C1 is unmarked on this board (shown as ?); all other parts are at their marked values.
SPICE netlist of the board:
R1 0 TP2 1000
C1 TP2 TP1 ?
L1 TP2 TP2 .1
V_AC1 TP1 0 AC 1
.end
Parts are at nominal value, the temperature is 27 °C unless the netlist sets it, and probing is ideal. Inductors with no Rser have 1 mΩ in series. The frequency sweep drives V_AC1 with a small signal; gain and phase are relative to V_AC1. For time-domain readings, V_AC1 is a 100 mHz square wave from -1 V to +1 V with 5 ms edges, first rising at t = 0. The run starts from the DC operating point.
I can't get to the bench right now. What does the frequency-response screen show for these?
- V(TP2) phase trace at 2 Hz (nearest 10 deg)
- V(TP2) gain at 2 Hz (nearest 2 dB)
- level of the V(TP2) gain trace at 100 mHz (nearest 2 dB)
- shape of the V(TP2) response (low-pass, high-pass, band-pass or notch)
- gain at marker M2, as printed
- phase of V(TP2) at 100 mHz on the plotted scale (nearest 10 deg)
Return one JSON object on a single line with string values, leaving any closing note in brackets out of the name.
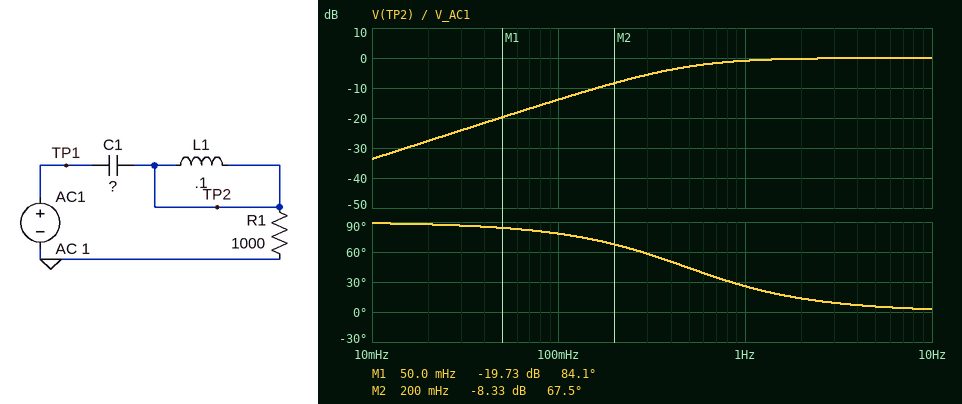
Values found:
{"V(TP2) phase trace at 2 Hz": "10 deg", "V(TP2) gain at 2 Hz": "0 dB", "level of the V(TP2) gain trace at 100 mHz": "-14 dB", "shape of the V(TP2) response": "high-pass", "gain at marker M2, as printed": "-8.33 dB", "phase of V(TP2) at 100 mHz on the plotted scale": "80 deg"}
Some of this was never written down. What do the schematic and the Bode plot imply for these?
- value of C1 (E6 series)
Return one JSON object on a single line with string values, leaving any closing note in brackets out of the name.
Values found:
{"value of C1": "330 µF"}
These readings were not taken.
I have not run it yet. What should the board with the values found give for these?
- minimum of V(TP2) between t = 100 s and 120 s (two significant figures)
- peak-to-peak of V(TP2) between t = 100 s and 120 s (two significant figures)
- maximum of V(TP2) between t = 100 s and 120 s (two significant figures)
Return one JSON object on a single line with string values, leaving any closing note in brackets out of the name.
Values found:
{"minimum of V(TP2) between t = 100 s and 120 s": "-2.0 V", "peak-to-peak of V(TP2) between t = 100 s and 120 s": "4.0 V", "maximum of V(TP2) between t = 100 s and 120 s": "2.0 V"}
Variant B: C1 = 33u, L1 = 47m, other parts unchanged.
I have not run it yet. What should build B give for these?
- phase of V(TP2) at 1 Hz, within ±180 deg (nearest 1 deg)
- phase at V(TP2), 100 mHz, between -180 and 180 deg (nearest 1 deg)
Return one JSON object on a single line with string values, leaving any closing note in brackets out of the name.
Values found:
{"phase of V(TP2) at 1 Hz, within ±180 deg": "78 deg", "phase at V(TP2), 100 mHz, between -180 and 180 deg": "89 deg"}
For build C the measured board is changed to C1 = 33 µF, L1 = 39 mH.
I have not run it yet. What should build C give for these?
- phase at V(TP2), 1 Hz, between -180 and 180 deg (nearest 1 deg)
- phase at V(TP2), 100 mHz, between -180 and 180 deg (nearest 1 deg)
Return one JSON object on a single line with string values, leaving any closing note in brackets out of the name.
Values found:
{"phase at V(TP2), 1 Hz, between -180 and 180 deg": "78 deg", "phase at V(TP2), 100 mHz, between -180 and 180 deg": "89 deg"}
